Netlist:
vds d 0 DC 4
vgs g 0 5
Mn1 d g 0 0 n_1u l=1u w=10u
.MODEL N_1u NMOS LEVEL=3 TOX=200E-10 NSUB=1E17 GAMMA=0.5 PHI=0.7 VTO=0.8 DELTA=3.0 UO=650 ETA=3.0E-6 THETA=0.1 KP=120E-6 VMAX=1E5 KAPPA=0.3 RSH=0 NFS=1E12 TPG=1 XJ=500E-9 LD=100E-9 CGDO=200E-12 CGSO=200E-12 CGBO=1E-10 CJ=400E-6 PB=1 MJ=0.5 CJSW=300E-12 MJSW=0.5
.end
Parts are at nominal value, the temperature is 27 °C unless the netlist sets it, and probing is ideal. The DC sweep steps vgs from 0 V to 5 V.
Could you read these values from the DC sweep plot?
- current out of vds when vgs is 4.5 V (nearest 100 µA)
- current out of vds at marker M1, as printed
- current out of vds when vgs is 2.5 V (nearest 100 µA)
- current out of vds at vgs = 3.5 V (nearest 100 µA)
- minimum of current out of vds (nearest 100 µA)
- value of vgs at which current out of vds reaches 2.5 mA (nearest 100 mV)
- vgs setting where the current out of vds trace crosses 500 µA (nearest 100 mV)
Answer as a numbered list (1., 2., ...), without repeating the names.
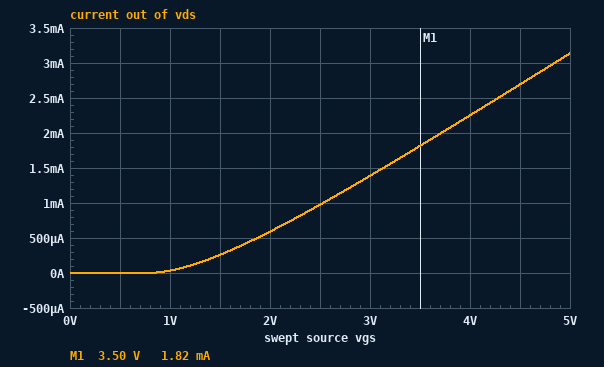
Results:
1. 2.7 mA
2. 1.82 mA
3. 1.0 mA
4. 1.8 mA
5. 0 A
6. 4.3 V
7. 1.9 V
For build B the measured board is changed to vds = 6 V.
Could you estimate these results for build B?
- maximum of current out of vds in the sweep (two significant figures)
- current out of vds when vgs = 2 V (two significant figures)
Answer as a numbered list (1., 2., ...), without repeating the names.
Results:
1. 3.3 mA
2. 620 µA
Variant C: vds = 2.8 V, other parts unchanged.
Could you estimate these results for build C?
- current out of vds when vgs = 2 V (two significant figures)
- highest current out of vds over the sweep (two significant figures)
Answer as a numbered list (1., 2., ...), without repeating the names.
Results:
1. 570 µA
2. 3.0 mA
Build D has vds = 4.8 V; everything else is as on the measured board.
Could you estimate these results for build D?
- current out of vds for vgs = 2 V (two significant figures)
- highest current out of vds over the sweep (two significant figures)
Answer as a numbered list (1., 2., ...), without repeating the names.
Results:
1. 600 µA
2. 3.2 mA
